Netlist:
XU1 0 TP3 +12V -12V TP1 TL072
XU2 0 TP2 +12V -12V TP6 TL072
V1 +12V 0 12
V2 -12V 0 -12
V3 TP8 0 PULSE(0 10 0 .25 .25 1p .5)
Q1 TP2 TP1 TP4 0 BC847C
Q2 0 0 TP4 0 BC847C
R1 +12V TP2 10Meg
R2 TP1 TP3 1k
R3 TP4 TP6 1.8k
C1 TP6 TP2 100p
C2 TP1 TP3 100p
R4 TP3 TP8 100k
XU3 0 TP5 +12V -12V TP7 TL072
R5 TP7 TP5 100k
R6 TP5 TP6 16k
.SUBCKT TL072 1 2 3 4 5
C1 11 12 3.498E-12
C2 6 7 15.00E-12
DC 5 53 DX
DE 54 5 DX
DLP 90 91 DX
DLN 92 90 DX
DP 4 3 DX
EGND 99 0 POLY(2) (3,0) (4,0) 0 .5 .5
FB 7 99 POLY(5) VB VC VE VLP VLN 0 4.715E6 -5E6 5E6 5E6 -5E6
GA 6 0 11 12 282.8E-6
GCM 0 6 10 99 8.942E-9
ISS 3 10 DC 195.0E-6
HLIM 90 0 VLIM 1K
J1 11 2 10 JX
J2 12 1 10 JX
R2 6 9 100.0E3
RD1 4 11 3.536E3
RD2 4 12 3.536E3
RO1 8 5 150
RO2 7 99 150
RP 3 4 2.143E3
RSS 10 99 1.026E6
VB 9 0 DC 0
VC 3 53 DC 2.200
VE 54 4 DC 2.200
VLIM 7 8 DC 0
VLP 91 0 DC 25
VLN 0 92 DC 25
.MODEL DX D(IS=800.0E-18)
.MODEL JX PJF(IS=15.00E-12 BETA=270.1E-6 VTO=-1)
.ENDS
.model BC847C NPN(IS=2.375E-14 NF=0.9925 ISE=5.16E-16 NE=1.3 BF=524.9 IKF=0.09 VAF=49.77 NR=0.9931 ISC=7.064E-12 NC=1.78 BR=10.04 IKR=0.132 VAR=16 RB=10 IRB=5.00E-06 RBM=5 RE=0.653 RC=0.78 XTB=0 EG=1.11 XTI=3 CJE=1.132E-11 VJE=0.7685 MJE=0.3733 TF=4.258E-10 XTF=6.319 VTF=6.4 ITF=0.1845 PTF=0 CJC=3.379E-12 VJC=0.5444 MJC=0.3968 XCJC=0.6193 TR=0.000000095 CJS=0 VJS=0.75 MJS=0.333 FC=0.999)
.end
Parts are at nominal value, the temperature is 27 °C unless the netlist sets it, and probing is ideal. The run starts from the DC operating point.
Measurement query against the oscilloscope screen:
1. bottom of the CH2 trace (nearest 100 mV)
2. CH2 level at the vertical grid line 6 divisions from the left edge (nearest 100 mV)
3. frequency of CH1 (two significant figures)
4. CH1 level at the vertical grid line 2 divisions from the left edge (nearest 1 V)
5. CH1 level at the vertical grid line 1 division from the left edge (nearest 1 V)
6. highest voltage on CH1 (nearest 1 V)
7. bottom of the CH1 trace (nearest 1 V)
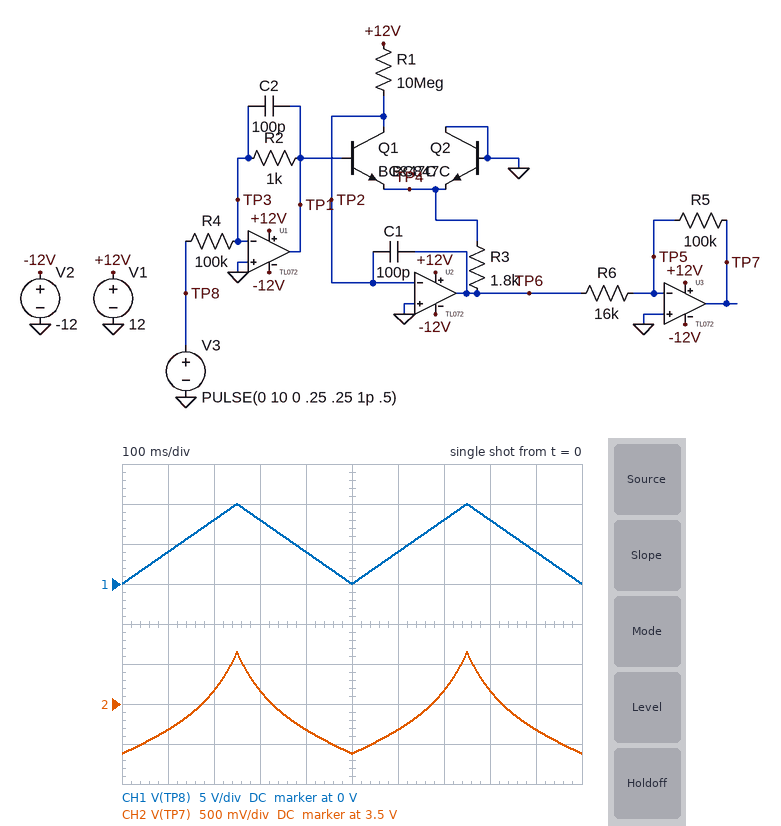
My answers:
2.9 V
3.2 V
2.0 Hz
8 V
4 V
10 V
0 V
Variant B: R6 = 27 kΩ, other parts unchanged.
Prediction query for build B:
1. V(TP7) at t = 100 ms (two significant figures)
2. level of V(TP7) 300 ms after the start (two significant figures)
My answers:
1.9 V
2.2 V
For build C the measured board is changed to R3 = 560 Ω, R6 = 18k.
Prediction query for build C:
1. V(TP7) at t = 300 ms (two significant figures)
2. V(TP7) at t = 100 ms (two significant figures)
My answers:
3.1 V
2.8 V
